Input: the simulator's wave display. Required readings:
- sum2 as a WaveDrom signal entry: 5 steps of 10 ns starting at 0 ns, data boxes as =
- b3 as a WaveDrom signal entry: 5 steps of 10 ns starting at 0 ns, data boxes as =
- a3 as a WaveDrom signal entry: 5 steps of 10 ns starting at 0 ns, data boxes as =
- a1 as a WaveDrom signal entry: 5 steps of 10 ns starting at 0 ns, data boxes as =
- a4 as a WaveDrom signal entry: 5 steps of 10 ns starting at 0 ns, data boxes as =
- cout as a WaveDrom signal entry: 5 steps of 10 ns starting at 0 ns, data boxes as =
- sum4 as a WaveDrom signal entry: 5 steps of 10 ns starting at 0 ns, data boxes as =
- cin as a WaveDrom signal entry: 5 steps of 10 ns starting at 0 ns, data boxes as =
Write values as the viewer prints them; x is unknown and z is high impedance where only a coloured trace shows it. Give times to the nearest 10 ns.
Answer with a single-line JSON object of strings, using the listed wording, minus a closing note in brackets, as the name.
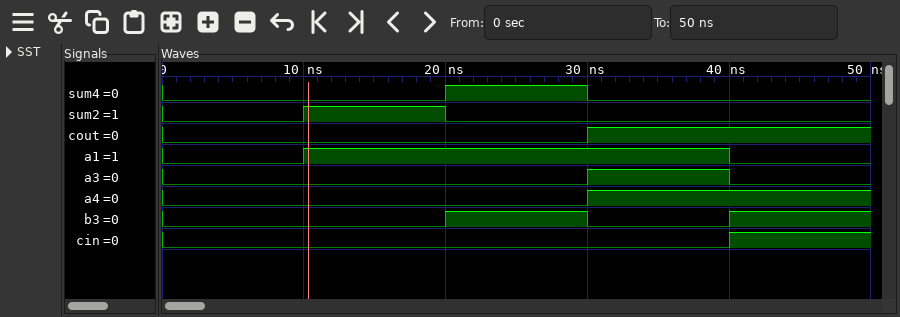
{"sum2 as a WaveDrom signal entry: 5 steps of 10 ns starting at 0 ns, data boxes as =": "{name: 'sum2', wave: '010..'}", "b3 as a WaveDrom signal entry: 5 steps of 10 ns starting at 0 ns, data boxes as =": "{name: 'b3', wave: '0.101'}", "a3 as a WaveDrom signal entry: 5 steps of 10 ns starting at 0 ns, data boxes as =": "{name: 'a3', wave: '0..10'}", "a1 as a WaveDrom signal entry: 5 steps of 10 ns starting at 0 ns, data boxes as =": "{name: 'a1', wave: '01..0'}", "a4 as a WaveDrom signal entry: 5 steps of 10 ns starting at 0 ns, data boxes as =": "{name: 'a4', wave: '0..1.'}", "cout as a WaveDrom signal entry: 5 steps of 10 ns starting at 0 ns, data boxes as =": "{name: 'cout', wave: '0..1.'}", "sum4 as a WaveDrom signal entry: 5 steps of 10 ns starting at 0 ns, data boxes as =": "{name: 'sum4', wave: '0.10.'}", "cin as a WaveDrom signal entry: 5 steps of 10 ns starting at 0 ns, data boxes as =": "{name: 'cin', wave: '0...1'}"}
